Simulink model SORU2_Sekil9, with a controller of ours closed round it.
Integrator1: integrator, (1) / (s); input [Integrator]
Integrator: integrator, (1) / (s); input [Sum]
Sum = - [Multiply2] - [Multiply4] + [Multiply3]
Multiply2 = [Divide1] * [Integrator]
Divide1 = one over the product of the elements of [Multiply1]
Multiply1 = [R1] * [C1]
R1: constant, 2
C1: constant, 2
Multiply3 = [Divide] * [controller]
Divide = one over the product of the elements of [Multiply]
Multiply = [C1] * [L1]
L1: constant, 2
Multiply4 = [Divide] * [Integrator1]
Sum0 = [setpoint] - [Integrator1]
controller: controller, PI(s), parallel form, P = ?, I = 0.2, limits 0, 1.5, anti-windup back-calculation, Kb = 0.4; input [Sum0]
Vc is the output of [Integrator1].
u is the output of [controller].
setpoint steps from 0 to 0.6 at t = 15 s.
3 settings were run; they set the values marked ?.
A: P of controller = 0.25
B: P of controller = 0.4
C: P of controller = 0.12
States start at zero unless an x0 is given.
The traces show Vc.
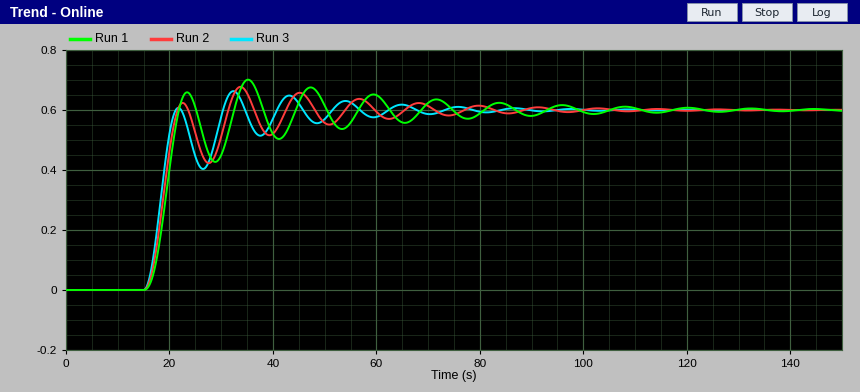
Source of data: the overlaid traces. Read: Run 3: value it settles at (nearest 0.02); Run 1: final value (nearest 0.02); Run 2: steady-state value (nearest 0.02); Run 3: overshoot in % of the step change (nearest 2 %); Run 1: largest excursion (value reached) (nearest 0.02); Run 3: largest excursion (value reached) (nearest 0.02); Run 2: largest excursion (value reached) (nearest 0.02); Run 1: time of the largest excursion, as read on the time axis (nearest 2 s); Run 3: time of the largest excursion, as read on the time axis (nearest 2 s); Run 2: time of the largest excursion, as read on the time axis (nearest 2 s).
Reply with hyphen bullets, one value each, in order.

- 0.60
- 0.60
- 0.60
- 10 %
- 0.70
- 0.66
- 0.68
- 36 s
- 32 s
- 34 s
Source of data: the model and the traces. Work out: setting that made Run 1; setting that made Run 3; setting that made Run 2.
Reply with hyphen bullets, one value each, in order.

- C
- B
- A
